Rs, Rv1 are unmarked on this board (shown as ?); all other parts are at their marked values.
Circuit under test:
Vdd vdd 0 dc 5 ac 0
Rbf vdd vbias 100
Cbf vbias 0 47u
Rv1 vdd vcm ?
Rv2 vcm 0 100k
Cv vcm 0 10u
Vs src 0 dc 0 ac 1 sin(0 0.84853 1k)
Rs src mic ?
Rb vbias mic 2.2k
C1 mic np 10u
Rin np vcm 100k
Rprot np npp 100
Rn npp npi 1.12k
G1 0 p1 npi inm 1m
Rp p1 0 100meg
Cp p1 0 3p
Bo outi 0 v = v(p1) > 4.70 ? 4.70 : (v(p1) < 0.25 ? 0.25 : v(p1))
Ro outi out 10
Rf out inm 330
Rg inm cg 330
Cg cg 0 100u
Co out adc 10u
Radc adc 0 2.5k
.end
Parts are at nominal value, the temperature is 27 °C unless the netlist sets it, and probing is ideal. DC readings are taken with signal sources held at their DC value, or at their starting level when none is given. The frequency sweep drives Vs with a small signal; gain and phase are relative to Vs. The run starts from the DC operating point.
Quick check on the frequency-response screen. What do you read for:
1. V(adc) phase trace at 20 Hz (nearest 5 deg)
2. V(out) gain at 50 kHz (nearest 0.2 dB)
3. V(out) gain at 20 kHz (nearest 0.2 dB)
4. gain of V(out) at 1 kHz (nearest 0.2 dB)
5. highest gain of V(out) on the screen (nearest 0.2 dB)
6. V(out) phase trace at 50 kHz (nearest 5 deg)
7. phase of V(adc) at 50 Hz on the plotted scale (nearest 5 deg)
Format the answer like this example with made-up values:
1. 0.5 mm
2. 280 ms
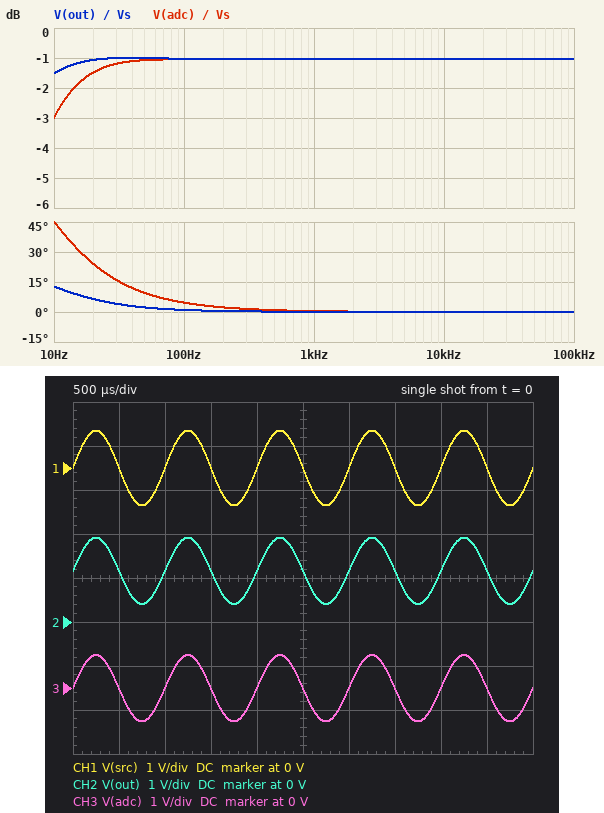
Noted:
1. 25 deg
2. -1.0 dB
3. -1.0 dB
4. -1.0 dB
5. -1.0 dB
6. 0 deg
7. 10 deg
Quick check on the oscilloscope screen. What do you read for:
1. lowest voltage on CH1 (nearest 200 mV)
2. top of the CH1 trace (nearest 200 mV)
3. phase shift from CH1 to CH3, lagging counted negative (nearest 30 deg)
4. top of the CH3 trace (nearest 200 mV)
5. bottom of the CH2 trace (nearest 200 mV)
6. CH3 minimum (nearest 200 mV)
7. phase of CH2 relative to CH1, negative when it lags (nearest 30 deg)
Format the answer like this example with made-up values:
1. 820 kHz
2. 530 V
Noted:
1. -800 mV
2. 800 mV
3. 0 deg
4. 800 mV
5. 400 mV
6. -800 mV
7. 0 deg
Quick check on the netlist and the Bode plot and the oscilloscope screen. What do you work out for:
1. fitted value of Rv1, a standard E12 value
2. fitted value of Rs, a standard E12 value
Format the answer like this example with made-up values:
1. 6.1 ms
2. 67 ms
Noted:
1. 330 kΩ
2. 2.7 kΩ
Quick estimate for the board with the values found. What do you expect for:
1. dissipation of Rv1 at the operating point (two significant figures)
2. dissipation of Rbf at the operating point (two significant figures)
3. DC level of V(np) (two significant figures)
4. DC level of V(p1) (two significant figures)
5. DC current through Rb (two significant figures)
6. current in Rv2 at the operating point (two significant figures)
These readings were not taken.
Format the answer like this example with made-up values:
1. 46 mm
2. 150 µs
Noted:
1. 45 µW
2. 100 µW
3. 1.2 V
4. 1.2 V
5. 1.0 mA
6. 12 µA
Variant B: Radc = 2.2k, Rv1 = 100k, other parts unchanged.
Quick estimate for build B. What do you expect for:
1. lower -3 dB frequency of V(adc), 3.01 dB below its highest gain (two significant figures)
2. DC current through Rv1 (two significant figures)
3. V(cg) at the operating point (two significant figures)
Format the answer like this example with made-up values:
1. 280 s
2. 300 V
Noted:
1. 8.6 Hz
2. 25 µA
3. 2.5 V
